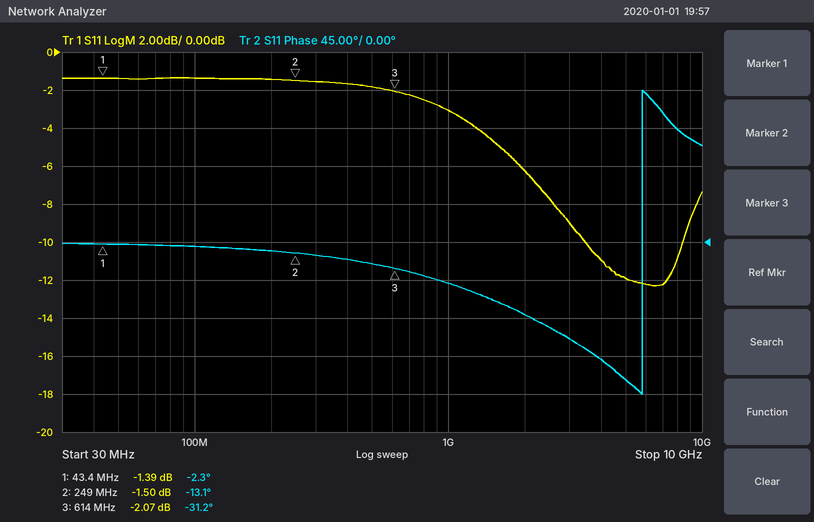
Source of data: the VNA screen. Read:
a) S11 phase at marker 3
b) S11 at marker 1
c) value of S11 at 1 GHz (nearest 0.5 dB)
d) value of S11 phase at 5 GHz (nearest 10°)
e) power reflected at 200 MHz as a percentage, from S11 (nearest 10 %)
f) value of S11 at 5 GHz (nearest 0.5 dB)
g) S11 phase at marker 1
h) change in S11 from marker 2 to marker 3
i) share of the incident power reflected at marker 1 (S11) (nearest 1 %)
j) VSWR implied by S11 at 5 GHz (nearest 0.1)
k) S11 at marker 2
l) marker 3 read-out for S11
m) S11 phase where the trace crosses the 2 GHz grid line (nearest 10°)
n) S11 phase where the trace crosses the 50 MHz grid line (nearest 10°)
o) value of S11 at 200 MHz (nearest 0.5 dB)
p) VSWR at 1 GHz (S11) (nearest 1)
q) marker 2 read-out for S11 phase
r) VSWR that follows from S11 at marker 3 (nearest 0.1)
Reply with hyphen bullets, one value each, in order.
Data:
- -31.2°
- -1.39 dB
- -3.0 dB
- -160°
- 70 %
- -12.0 dB
- -2.3°
- -0.57 dB
- 73 %
- 1.7
- -1.50 dB
- -2.07 dB
- -90°
- 0°
- -1.5 dB
- 6
- -13.1°
- 8.4
